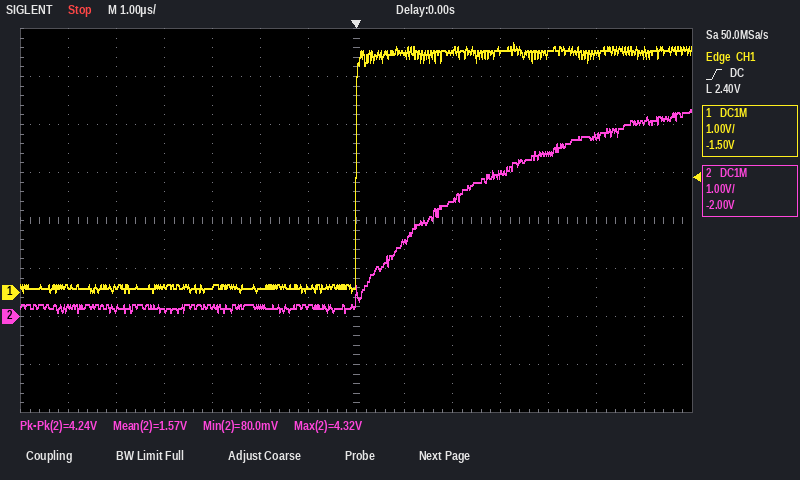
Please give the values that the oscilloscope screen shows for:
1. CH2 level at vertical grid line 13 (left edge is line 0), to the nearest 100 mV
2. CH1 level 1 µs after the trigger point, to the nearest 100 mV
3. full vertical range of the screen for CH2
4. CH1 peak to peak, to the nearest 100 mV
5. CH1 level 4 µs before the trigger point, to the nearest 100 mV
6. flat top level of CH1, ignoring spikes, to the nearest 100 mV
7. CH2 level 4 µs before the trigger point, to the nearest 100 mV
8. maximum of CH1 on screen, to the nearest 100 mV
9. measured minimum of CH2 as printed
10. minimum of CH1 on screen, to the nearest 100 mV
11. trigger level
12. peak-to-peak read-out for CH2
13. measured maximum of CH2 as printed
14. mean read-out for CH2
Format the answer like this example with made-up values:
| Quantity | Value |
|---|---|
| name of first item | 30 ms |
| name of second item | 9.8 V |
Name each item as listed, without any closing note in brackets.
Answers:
| Quantity | Value |
|---|---|
| CH2 level at vertical grid line 13 (left edge is line 0), to the nearest 100 mV | 4.0 V |
| CH1 level 1 µs after the trigger point, to the nearest 100 mV | 5.0 V |
| full vertical range of the screen for CH2 | 8 V |
| CH1 peak to peak, to the nearest 100 mV | 5.2 V |
| CH1 level 4 µs before the trigger point, to the nearest 100 mV | 100 mV |
| flat top level of CH1, ignoring spikes, to the nearest 100 mV | 5.0 V |
| CH2 level 4 µs before the trigger point, to the nearest 100 mV | 100 mV |
| maximum of CH1 on screen, to the nearest 100 mV | 5.2 V |
| measured minimum of CH2 as printed | 80.0 mV |
| minimum of CH1 on screen, to the nearest 100 mV | 0.0 V |
| trigger level | 2.40 V |
| peak-to-peak read-out for CH2 | 4.24 V |
| measured maximum of CH2 as printed | 4.32 V |
| mean read-out for CH2 | 1.57 V |
